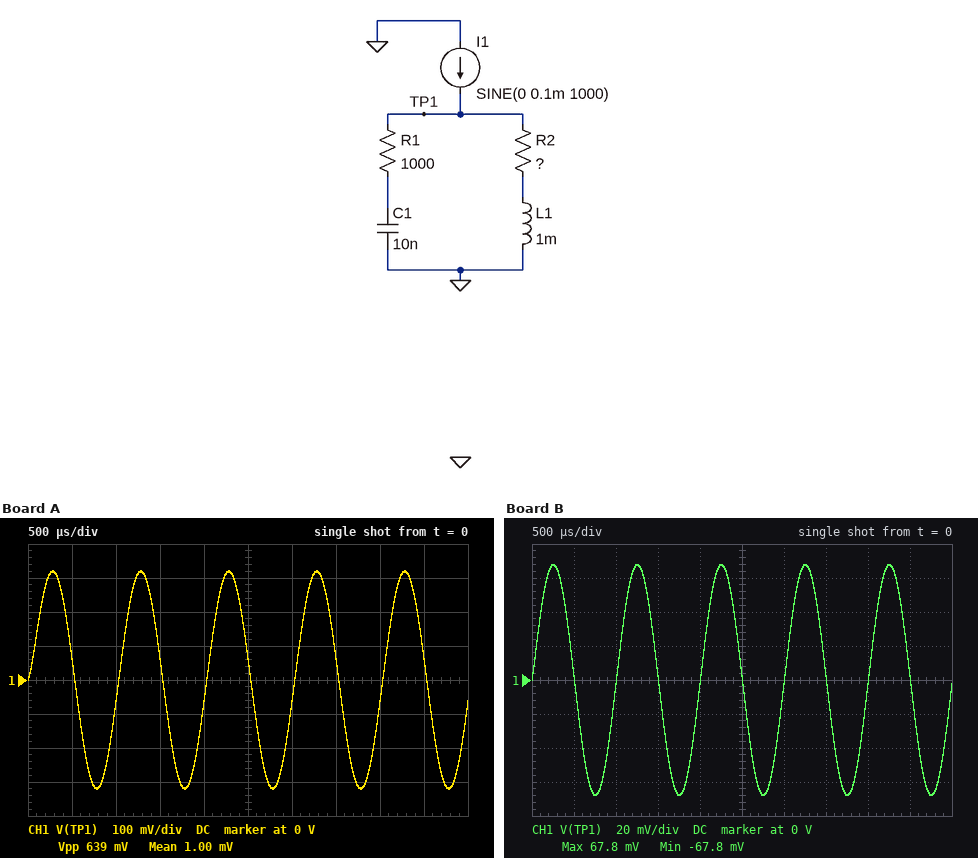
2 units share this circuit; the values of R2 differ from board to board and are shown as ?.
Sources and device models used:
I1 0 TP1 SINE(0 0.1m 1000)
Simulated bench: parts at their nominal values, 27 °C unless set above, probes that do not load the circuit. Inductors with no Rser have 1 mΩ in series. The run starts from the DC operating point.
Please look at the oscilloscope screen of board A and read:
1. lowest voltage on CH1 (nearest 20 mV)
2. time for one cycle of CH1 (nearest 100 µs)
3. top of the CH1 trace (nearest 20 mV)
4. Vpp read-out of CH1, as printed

-320 mV
1.0 ms
320 mV
639 mV
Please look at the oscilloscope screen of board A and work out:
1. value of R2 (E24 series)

3.3 kΩ
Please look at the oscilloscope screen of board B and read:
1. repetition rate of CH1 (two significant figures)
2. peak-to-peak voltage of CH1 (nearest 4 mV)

1.0 kHz
136 mV
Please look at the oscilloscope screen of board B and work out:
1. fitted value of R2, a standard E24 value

680 Ω
